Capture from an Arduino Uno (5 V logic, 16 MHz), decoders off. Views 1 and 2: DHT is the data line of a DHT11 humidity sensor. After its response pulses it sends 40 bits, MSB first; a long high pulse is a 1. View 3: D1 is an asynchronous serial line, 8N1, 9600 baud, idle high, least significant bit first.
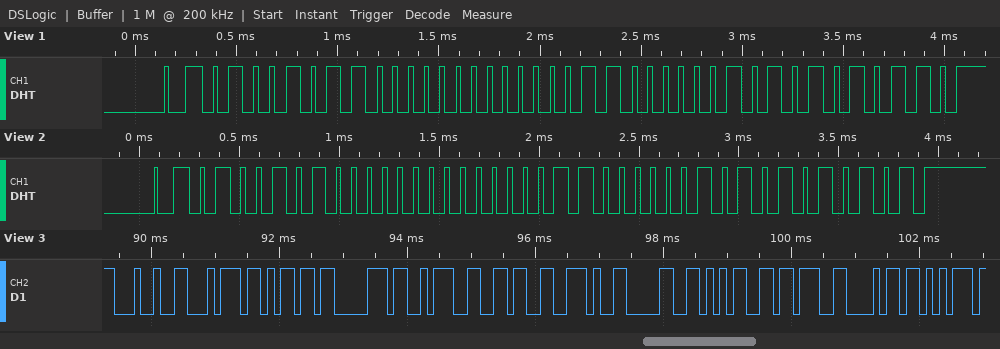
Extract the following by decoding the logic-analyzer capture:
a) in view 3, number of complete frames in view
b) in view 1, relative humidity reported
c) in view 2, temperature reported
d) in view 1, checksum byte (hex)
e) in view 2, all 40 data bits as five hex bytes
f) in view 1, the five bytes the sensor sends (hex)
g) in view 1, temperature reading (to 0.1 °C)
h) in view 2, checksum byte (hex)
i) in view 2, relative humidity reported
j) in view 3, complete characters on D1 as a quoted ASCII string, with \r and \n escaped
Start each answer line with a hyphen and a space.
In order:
- 12
- 75 %
- 6.5 °C
- 0x56
- 4A 00 06 05 55
- 4B 00 06 05 56
- 6.5 °C
- 0x55
- 74 %
- "$tmp:6.05;hu"
